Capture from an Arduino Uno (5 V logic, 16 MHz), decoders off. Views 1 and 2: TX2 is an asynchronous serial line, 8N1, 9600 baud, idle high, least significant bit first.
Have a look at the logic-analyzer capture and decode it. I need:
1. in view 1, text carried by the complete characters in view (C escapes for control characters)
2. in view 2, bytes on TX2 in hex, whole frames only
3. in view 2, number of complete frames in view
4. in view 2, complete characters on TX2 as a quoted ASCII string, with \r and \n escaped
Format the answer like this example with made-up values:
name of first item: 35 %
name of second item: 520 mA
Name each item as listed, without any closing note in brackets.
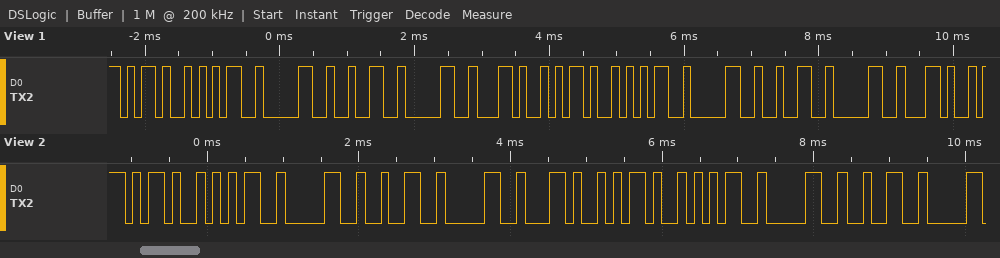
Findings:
in view 1, text carried by the complete characters in view: "-5020,-5020,"
in view 2, bytes on TX2 in hex, whole frames only: 2D 35 30 32 30 2C 2D 35 30 32
in view 2, number of complete frames in view: 10
in view 2, complete characters on TX2 as a quoted ASCII string, with \r and \n escaped: "-5020,-502"
